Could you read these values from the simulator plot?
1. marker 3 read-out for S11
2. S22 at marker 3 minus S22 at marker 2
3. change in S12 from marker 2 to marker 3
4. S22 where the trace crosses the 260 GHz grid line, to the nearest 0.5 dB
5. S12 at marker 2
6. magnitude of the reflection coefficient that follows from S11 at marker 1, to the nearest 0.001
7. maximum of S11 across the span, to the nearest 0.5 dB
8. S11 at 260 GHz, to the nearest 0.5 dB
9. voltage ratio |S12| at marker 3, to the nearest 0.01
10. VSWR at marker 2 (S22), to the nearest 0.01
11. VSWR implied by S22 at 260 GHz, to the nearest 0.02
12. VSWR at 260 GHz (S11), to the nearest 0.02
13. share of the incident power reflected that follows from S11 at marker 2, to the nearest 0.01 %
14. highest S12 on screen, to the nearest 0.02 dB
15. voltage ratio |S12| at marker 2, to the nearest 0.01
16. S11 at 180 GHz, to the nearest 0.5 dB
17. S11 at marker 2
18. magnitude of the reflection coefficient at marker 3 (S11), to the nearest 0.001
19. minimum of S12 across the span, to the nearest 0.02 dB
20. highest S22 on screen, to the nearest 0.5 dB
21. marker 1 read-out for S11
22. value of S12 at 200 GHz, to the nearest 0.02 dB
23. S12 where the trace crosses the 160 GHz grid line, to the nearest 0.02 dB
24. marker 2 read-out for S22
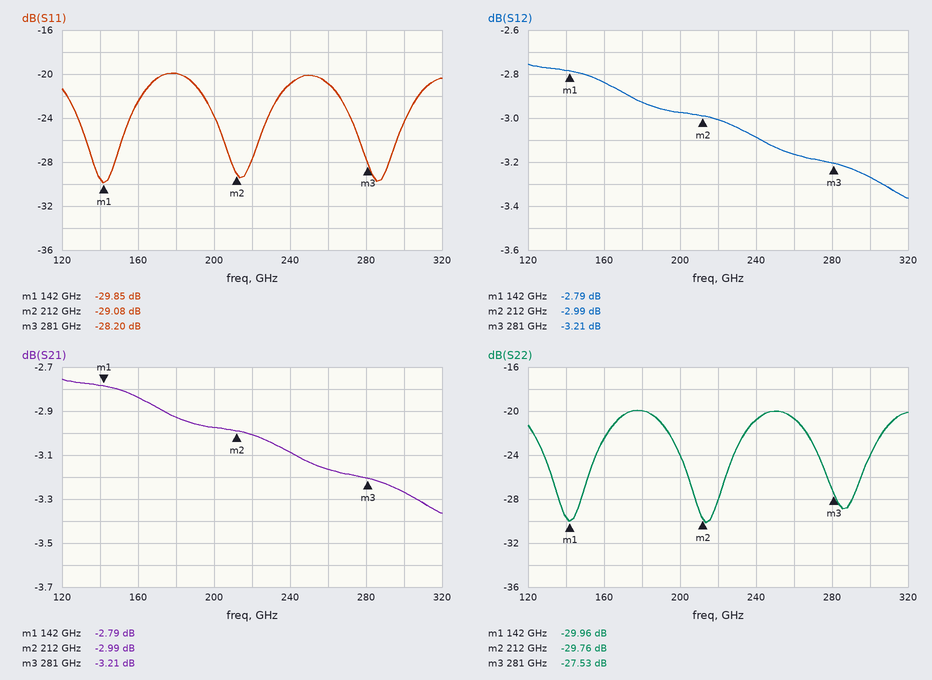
-28.20 dB
2.23 dB
-0.22 dB
-20.5 dB
-2.99 dB
0.032
-20.0 dB
-21.0 dB
0.69
1.07
1.20
1.20
0.12 %
-2.76 dB
0.71
-20.0 dB
-29.08 dB
0.039
-3.36 dB
-20.0 dB
-29.85 dB
-2.98 dB
-2.84 dB
-29.76 dB
